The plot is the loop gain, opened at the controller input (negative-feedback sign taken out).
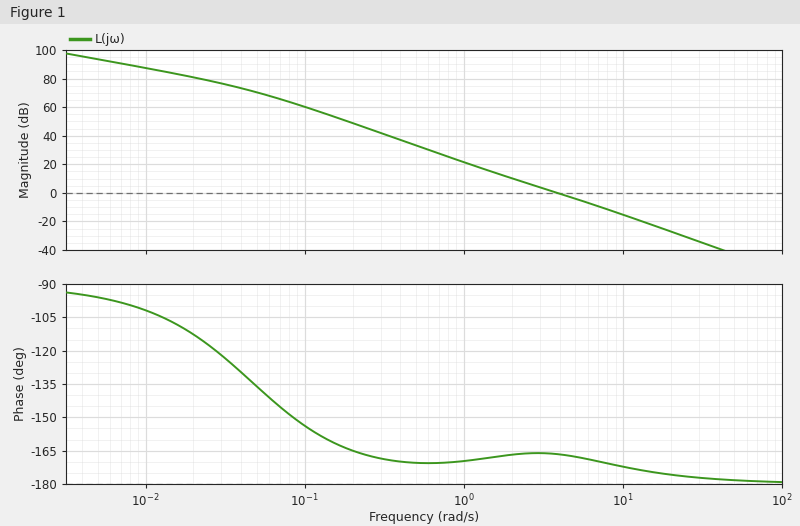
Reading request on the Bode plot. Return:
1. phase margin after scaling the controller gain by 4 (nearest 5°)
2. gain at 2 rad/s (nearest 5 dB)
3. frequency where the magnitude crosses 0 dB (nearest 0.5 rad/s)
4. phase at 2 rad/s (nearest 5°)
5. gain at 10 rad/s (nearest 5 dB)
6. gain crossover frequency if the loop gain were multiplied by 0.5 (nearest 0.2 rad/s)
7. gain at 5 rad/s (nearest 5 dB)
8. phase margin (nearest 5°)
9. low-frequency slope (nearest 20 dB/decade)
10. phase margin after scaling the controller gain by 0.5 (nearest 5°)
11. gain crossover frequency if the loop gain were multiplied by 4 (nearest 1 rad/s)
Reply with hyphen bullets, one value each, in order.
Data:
- 10°
- 10 dB
- 4.0 rad/s
- -165°
- -15 dB
- 2.6 rad/s
- -5 dB
- 15°
- -20 dB/decade
- 15°
- 8 rad/s
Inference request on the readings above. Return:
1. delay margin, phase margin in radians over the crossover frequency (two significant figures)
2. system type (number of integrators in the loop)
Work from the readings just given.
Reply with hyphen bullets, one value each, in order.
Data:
- 0.065 s
- 1
